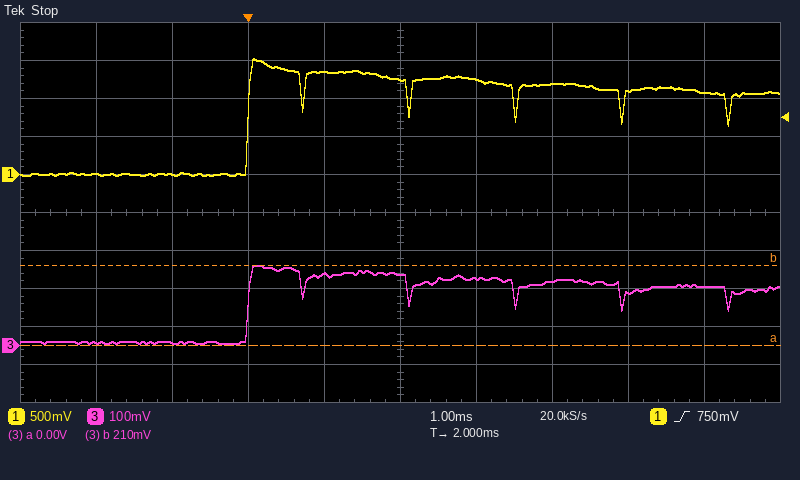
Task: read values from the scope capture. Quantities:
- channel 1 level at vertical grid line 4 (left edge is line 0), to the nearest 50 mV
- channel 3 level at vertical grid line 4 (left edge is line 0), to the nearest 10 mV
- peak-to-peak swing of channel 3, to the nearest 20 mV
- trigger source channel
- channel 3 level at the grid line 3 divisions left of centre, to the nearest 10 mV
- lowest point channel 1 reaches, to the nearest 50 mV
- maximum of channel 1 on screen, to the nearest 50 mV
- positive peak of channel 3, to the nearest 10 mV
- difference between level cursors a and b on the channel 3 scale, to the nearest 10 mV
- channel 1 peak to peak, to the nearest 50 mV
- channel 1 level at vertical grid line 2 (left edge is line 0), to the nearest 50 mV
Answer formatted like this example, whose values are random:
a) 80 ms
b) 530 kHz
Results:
a) 1.35 V
b) 190 mV
c) 200 mV
d) channel 1
e) 10 mV
f) 0 mV
g) 1.55 V
h) 210 mV
i) 210 mV
j) 1.55 V
k) 0 mV
